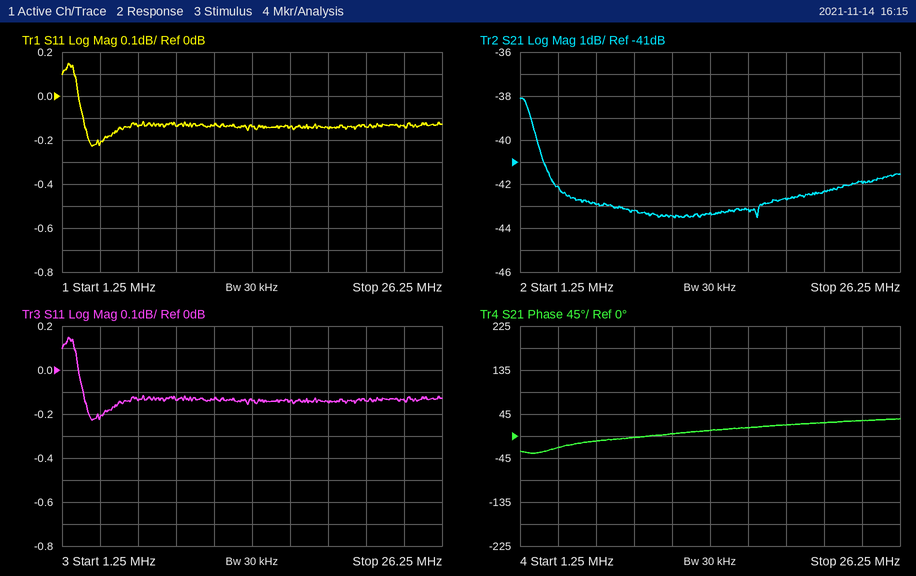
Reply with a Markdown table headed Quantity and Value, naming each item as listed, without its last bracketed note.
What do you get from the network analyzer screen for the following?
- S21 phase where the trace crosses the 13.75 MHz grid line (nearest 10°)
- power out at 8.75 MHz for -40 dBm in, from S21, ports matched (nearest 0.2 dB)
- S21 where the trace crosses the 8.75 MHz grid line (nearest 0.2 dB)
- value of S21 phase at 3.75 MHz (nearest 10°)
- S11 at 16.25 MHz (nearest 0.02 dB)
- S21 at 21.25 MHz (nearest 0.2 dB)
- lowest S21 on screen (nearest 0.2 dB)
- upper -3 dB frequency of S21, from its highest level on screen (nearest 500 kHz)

| Quantity | Value |
|---|---|
| S21 phase where the trace crosses the 13.75 MHz grid line | 10° |
| power out at 8.75 MHz for -40 dBm in, from S21, ports matched | -83.2 dBm |
| S21 where the trace crosses the 8.75 MHz grid line | -43.2 dB |
| value of S21 phase at 3.75 MHz | -20° |
| S11 at 16.25 MHz | -0.14 dB |
| S21 at 21.25 MHz | -42.4 dB |
| lowest S21 on screen | -43.6 dB |
| upper -3 dB frequency of S21, from its highest level on screen | 3.0 MHz |
